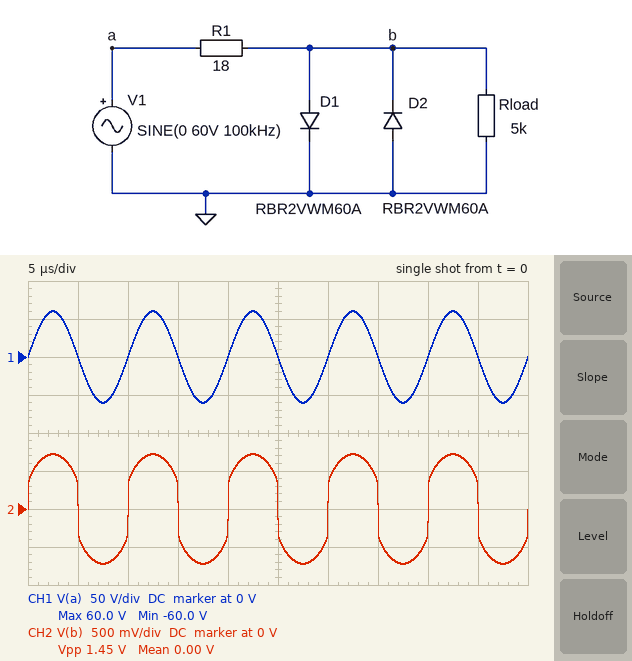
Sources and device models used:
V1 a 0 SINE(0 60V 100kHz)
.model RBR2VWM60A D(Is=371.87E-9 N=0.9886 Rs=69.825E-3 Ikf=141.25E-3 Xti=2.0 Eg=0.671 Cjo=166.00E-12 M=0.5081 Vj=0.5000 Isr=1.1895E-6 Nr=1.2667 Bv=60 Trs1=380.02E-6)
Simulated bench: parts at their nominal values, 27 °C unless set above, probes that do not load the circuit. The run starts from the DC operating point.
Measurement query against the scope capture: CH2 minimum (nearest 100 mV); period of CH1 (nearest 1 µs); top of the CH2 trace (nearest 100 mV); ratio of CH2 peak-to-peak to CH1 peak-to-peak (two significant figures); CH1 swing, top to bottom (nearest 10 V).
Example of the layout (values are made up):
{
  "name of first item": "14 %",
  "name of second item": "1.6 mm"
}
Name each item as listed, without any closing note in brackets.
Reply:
{
  "CH2 minimum": "-700 mV",
  "period of CH1": "10 µs",
  "top of the CH2 trace": "700 mV",
  "ratio of CH2 peak-to-peak to CH1 peak-to-peak": "0.012",
  "CH1 swing, top to bottom": "120 V"
}
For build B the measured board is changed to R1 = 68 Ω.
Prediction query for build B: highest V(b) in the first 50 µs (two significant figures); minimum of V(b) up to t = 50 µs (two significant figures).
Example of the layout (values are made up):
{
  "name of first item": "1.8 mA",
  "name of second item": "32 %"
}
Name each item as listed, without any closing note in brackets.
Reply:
{
  "highest V(b) in the first 50 µs": "490 mV",
  "minimum of V(b) up to t = 50 µs": "-490 mV"
}
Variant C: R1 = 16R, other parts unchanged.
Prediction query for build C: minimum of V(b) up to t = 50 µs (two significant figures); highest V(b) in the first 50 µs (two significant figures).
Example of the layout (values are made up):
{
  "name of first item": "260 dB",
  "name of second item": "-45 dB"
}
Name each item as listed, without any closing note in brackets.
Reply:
{
  "minimum of V(b) up to t = 50 µs": "-760 mV",
  "highest V(b) in the first 50 µs": "760 mV"
}
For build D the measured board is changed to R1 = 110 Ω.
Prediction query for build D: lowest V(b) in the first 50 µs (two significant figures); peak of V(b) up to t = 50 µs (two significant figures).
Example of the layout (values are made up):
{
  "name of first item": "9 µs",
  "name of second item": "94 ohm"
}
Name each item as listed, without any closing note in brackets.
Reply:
{
  "lowest V(b) in the first 50 µs": "-440 mV",
  "peak of V(b) up to t = 50 µs": "440 mV"
}
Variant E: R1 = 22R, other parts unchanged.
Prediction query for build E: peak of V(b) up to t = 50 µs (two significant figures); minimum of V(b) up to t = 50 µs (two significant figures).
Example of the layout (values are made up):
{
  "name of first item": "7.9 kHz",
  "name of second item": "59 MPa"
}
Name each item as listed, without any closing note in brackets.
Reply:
{
  "peak of V(b) up to t = 50 µs": "670 mV",
  "minimum of V(b) up to t = 50 µs": "-670 mV"
}
